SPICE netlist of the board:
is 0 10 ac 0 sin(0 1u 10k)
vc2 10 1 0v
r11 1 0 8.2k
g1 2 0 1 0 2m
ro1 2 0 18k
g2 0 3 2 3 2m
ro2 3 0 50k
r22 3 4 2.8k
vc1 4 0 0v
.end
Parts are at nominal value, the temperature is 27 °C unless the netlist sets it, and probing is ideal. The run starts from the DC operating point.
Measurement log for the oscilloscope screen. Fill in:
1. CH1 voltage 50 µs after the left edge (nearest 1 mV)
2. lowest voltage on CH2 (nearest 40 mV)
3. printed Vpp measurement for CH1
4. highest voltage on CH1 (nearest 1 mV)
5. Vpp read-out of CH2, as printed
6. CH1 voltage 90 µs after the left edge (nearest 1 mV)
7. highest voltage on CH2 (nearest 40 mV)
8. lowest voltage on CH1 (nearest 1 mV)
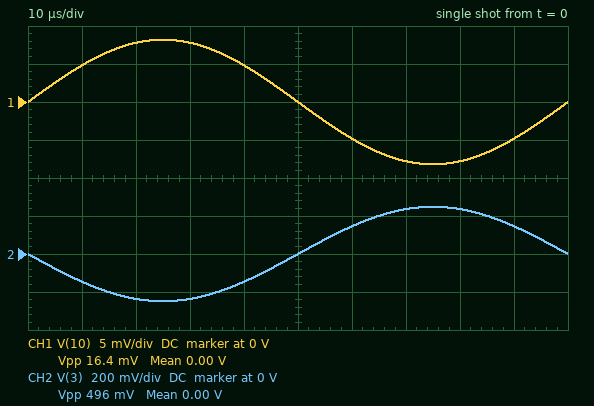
0 V
-240 mV
16.4 mV
8 mV
496 mV
-5 mV
240 mV
-8 mV
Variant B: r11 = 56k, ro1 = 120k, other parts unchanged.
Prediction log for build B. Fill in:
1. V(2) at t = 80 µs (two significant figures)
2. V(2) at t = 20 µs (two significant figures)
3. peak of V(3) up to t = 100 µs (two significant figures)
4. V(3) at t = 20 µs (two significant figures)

13 V
-13 V
11 V
-11 V
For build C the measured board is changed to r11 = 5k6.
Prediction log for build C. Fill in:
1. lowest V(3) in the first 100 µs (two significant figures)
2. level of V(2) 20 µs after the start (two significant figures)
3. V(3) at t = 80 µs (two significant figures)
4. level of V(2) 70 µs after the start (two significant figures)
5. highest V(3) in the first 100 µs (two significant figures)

-170 mV
-190 mV
160 mV
190 mV
170 mV
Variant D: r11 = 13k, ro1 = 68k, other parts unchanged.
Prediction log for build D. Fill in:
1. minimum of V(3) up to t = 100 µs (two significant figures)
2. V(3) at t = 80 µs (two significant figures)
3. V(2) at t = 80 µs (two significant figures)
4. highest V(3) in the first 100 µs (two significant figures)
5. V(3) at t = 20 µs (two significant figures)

-1.5 V
1.4 V
1.7 V
1.5 V
-1.4 V
